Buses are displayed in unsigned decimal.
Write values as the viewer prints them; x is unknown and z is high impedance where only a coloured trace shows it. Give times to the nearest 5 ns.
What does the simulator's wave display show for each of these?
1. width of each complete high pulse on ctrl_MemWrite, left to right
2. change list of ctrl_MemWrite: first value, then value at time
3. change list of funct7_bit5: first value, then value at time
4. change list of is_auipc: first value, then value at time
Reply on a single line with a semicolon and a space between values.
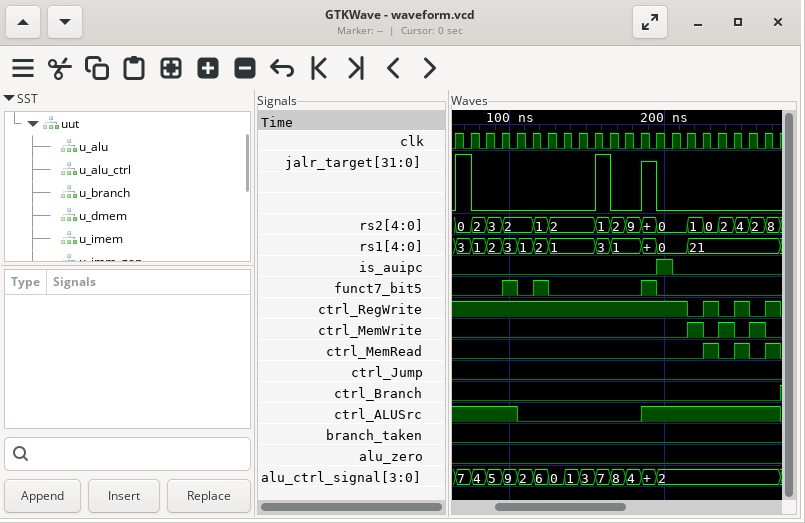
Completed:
10 ns, 10 ns, 10 ns; 0, 1 at 215 ns, 0 at 225 ns, 1 at 235 ns, 0 at 245 ns, 1 at 255 ns, 0 at 265 ns; 0, 1 at 95 ns, 0 at 105 ns, 1 at 115 ns, 0 at 125 ns, 1 at 185 ns, 0 at 195 ns; 0, 1 at 195 ns, 0 at 205 ns
